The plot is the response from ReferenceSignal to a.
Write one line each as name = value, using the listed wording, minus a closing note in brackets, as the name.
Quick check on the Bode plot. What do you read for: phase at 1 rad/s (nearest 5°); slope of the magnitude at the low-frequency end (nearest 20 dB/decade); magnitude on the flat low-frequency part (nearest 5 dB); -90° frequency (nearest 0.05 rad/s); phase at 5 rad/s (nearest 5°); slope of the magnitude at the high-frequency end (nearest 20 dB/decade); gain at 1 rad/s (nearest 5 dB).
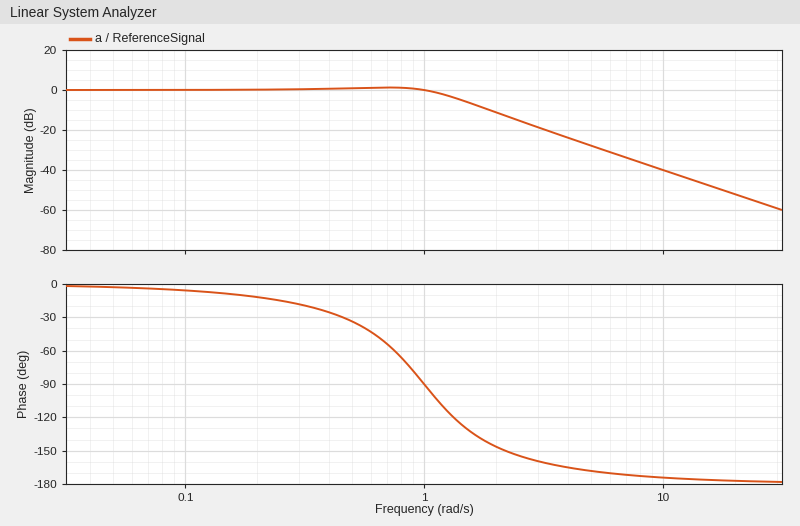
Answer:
phase at 1 rad/s = -90°
slope of the magnitude at the low-frequency end = 0 dB/decade
magnitude on the flat low-frequency part = 0 dB
-90° frequency = 1.00 rad/s
phase at 5 rad/s = -170°
slope of the magnitude at the high-frequency end = -40 dB/decade
gain at 1 rad/s = 0 dB
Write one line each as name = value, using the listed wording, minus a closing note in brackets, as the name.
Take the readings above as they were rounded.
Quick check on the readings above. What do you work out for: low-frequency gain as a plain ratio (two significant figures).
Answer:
low-frequency gain as a plain ratio = 1.0
